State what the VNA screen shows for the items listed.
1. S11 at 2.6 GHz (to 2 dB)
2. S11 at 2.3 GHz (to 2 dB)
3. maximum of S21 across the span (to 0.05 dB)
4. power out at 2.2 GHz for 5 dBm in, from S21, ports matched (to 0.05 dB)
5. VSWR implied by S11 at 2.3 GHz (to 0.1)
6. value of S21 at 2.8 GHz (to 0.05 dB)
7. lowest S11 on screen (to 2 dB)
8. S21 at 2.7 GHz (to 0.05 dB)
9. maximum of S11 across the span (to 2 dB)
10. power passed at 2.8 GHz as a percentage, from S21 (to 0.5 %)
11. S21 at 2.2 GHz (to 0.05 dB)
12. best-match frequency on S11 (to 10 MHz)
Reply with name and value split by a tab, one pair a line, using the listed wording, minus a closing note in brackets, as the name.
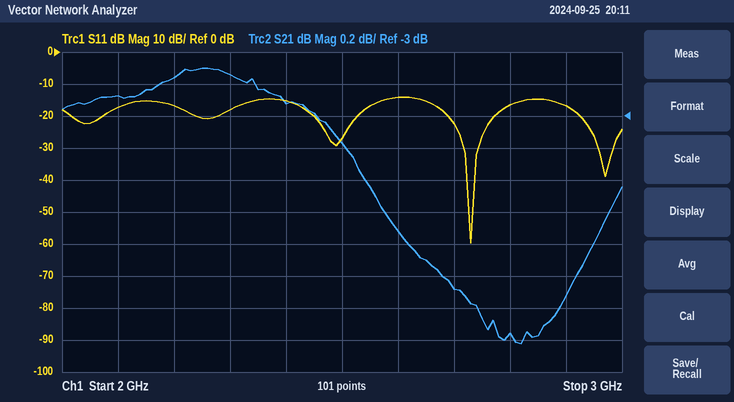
S11 at 2.6 GHz	-14 dB
S11 at 2.3 GHz	-18 dB
maximum of S21 across the span	-2.70 dB
power out at 2.2 GHz for 5 dBm in, from S21, ports matched	2.25 dBm
VSWR implied by S11 at 2.3 GHz	1.3
value of S21 at 2.8 GHz	-4.35 dB
lowest S11 on screen	-60 dB
S21 at 2.7 GHz	-4.10 dB
maximum of S11 across the span	-14 dB
power passed at 2.8 GHz as a percentage, from S21	36.5 %
S21 at 2.2 GHz	-2.75 dB
best-match frequency on S11	2.73 GHz
